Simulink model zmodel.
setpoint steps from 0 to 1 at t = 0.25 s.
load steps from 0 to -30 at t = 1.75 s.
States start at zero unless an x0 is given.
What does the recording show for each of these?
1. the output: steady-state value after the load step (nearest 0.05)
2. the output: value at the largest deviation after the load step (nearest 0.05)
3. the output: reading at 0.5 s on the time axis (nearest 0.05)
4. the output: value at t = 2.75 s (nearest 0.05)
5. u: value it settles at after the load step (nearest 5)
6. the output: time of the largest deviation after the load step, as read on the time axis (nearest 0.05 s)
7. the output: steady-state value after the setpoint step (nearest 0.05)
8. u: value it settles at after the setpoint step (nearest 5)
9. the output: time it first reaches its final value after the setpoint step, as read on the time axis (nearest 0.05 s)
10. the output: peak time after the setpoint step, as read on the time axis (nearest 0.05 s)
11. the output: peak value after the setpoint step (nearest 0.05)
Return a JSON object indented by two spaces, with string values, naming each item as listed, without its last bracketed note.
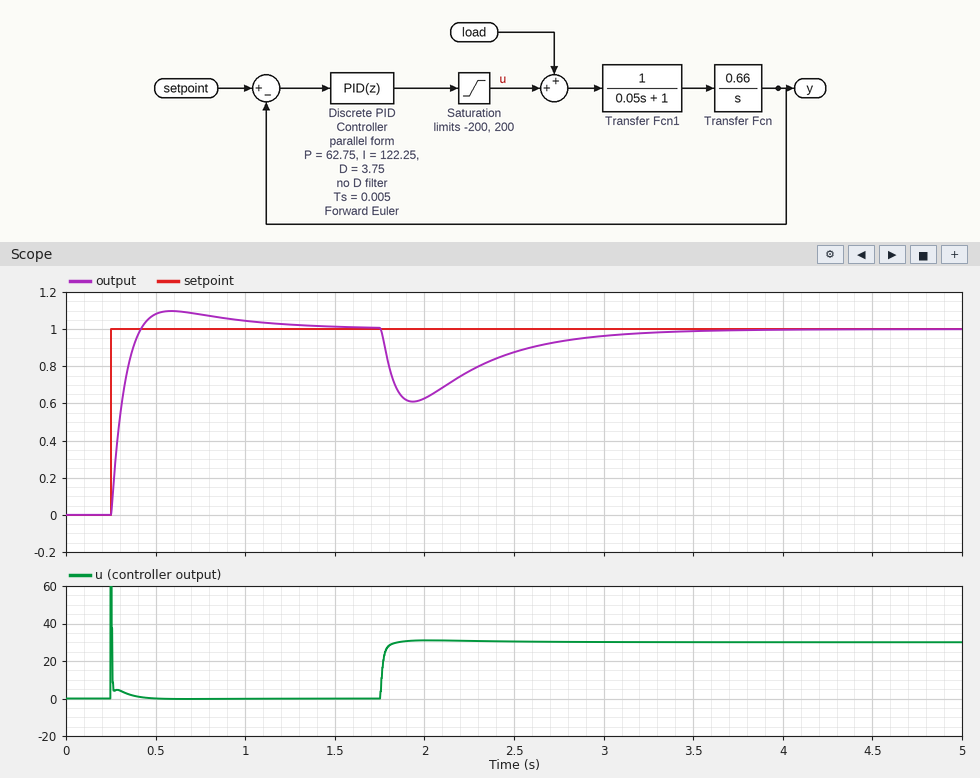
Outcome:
{
  "the output: steady-state value after the load step": "1.00",
  "the output: value at the largest deviation after the load step": "0.60",
  "the output: reading at 0.5 s on the time axis": "1.10",
  "the output: value at t = 2.75 s": "0.95",
  "u: value it settles at after the load step": "30",
  "the output: time of the largest deviation after the load step, as read on the time axis": "1.95 s",
  "the output: steady-state value after the setpoint step": "1.00",
  "u: value it settles at after the setpoint step": "0",
  "the output: time it first reaches its final value after the setpoint step, as read on the time axis": "0.40 s",
  "the output: peak time after the setpoint step, as read on the time axis": "0.60 s",
  "the output: peak value after the setpoint step": "1.10"
}
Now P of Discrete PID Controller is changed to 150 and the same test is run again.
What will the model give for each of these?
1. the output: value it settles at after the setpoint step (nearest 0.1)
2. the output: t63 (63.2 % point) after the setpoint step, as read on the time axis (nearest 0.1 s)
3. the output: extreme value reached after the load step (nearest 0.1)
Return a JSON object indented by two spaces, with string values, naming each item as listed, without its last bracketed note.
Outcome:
{
  "the output: value it settles at after the setpoint step": "1.0",
  "the output: t63 (63.2 % point) after the setpoint step, as read on the time axis": "0.3 s",
  "the output: extreme value reached after the load step": "0.8"
}
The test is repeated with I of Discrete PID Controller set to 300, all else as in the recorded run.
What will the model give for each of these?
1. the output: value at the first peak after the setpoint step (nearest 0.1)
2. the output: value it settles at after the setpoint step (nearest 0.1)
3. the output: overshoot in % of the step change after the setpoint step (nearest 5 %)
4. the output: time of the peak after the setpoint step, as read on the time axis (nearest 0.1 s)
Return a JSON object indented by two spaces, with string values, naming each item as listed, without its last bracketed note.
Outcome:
{
  "the output: value at the first peak after the setpoint step": "1.2",
  "the output: value it settles at after the setpoint step": "1.0",
  "the output: overshoot in % of the step change after the setpoint step": "20 %",
  "the output: time of the peak after the setpoint step, as read on the time axis": "0.5 s"
}
